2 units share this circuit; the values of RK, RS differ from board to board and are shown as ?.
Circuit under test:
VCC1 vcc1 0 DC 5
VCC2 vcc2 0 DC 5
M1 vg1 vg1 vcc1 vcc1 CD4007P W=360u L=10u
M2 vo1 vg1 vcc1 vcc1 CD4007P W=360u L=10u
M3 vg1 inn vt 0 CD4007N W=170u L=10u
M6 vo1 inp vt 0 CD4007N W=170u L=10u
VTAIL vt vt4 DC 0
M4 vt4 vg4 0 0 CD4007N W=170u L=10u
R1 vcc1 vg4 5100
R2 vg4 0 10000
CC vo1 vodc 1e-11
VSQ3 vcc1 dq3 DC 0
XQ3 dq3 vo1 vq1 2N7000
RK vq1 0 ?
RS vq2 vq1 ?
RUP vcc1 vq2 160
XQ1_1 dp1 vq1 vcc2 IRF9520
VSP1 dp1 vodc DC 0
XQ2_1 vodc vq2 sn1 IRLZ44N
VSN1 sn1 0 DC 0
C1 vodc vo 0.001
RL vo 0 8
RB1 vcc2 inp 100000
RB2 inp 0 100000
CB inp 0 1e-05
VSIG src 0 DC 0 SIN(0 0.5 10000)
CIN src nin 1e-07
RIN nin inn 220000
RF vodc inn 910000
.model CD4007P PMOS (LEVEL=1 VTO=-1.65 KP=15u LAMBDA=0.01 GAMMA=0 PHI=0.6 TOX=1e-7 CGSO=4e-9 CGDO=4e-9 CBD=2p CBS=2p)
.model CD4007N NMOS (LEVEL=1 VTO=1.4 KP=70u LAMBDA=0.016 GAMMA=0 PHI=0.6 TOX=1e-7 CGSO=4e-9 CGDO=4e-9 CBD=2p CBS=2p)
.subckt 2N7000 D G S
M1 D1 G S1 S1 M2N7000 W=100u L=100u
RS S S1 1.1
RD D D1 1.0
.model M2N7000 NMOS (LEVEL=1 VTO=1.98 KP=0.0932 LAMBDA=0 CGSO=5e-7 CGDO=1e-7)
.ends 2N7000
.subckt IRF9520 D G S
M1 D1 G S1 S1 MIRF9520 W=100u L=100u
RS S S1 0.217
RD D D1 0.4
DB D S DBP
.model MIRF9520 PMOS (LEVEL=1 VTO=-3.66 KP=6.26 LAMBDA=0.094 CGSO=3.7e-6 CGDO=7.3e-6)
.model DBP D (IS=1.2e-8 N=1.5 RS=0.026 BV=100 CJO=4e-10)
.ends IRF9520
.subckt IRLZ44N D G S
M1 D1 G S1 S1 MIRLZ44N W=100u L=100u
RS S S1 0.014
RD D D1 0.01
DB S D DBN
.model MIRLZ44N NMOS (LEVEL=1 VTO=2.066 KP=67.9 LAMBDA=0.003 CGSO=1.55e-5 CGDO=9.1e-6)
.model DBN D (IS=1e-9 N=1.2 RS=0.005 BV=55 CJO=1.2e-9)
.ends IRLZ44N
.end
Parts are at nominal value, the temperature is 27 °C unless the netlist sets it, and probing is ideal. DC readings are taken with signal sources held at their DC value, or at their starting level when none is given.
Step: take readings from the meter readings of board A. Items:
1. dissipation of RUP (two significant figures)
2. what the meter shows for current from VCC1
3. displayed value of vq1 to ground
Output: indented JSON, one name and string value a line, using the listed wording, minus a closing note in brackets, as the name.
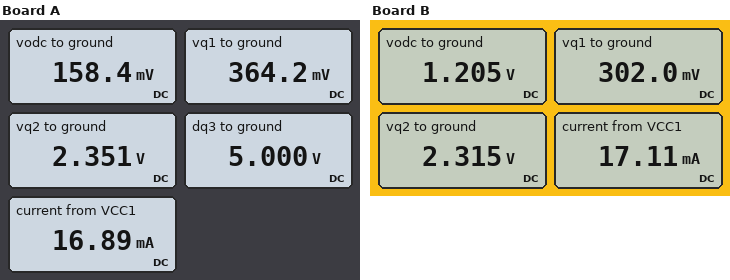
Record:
{
  "dissipation of RUP": "44 mW",
  "what the meter shows for current from VCC1": "16.89 mA",
  "displayed value of vq1 to ground": "364.2 mV"
}
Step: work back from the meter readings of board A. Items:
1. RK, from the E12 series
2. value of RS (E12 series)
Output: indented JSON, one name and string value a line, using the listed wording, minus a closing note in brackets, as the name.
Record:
{
  "RK, from the E12 series": "22 Ω",
  "value of RS": "120 Ω"
}
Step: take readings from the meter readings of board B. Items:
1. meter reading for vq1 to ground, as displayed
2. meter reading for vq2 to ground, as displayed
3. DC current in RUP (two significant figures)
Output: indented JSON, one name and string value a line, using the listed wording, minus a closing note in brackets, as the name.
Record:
{
  "meter reading for vq1 to ground, as displayed": "302.0 mV",
  "meter reading for vq2 to ground, as displayed": "2.315 V",
  "DC current in RUP": "17 mA"
}
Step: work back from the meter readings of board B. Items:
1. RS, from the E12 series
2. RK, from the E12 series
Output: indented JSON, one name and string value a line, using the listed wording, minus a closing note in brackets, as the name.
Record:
{
  "RS, from the E12 series": "120 Ω",
  "RK, from the E12 series": "18 Ω"
}
